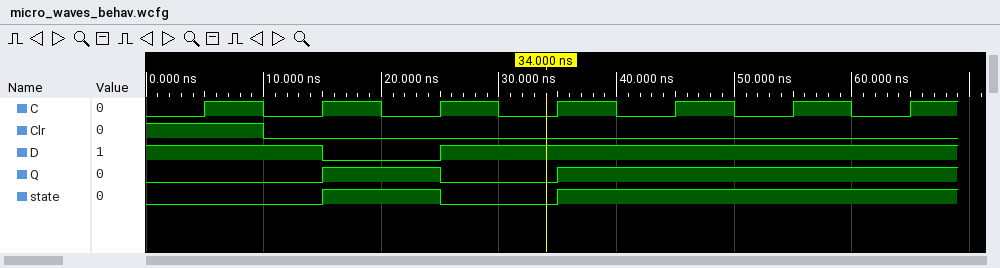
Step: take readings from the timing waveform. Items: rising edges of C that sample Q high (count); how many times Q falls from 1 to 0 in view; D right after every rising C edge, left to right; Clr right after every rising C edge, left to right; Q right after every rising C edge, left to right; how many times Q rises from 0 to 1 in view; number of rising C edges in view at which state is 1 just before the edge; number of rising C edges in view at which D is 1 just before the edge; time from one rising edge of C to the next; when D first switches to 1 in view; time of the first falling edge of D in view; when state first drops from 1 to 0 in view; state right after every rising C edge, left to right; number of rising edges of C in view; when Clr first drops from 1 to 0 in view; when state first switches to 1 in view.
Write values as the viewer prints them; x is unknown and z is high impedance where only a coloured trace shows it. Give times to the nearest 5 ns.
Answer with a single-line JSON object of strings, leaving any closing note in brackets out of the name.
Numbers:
{"rising edges of C that sample Q high": "4", "how many times Q falls from 1 to 0 in view": "1", "D right after every rising C edge, left to right": "1 0 1 1 1 1 1", "Clr right after every rising C edge, left to right": "1 0 0 0 0 0 0", "Q right after every rising C edge, left to right": "0 1 0 1 1 1 1", "how many times Q rises from 0 to 1 in view": "2", "number of rising C edges in view at which state is 1 just before the edge": "4", "number of rising C edges in view at which D is 1 just before the edge": "6", "time from one rising edge of C to the next": "10 ns", "when D first switches to 1 in view": "25 ns", "time of the first falling edge of D in view": "15 ns", "when state first drops from 1 to 0 in view": "25 ns", "state right after every rising C edge, left to right": "0 1 0 1 1 1 1", "number of rising edges of C in view": "7", "when Clr first drops from 1 to 0 in view": "10 ns", "when state first switches to 1 in view": "15 ns"}
